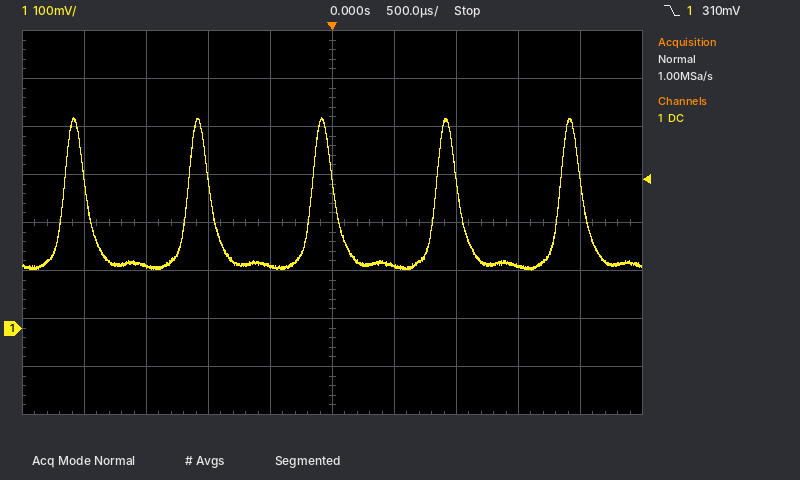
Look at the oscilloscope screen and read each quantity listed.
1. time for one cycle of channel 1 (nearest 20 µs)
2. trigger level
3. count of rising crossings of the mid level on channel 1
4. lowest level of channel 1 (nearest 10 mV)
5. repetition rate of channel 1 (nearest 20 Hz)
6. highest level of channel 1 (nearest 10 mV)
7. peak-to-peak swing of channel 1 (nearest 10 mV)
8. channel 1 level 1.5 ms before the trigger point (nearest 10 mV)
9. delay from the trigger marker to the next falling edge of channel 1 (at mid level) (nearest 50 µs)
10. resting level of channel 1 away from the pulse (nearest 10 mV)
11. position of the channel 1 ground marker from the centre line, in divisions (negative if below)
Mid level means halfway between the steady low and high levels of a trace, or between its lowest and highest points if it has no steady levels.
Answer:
1.00 ms
310 mV
5
120 mV
1.00 kHz
440 mV
320 mV
130 mV
1.00 ms
130 mV
-2.2 div
